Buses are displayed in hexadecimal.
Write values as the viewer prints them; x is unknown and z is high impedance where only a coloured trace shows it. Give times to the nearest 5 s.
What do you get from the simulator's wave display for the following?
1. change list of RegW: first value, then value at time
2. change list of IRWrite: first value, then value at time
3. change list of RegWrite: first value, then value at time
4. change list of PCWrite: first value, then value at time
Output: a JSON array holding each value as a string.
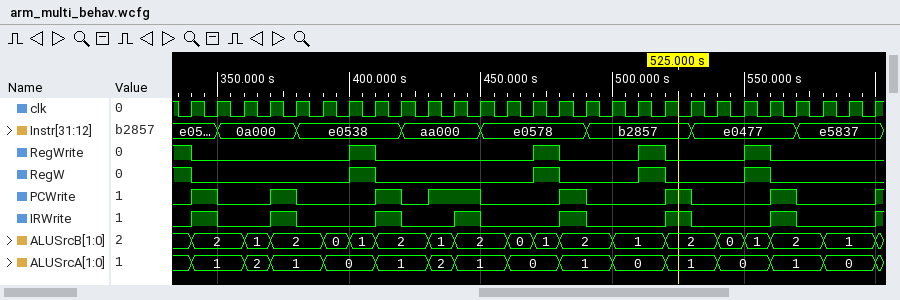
["1, 0 at 340 s, 1 at 400 s, 0 at 410 s, 1 at 470 s, 0 at 480 s, 1 at 510 s, 0 at 520 s, 1 at 550 s, 0 at 560 s", "0, 1 at 340 s, 0 at 350 s, 1 at 370 s, 0 at 380 s, 1 at 410 s, 0 at 420 s, 1 at 440 s, 0 at 450 s, 1 at 480 s, 0 at 490 s, 1 at 520 s, 0 at 530 s, 1 at 560 s, 0 at 570 s, 1 at 600 s", "1, 0 at 340 s, 1 at 400 s, 0 at 410 s, 1 at 470 s, 0 at 480 s, 1 at 510 s, 0 at 520 s, 1 at 550 s, 0 at 560 s", "0, 1 at 340 s, 0 at 350 s, 1 at 370 s, 0 at 380 s, 1 at 410 s, 0 at 420 s, 1 at 430 s, 0 at 450 s, 1 at 480 s, 0 at 490 s, 1 at 520 s, 0 at 530 s, 1 at 560 s, 0 at 570 s, 1 at 600 s"]
